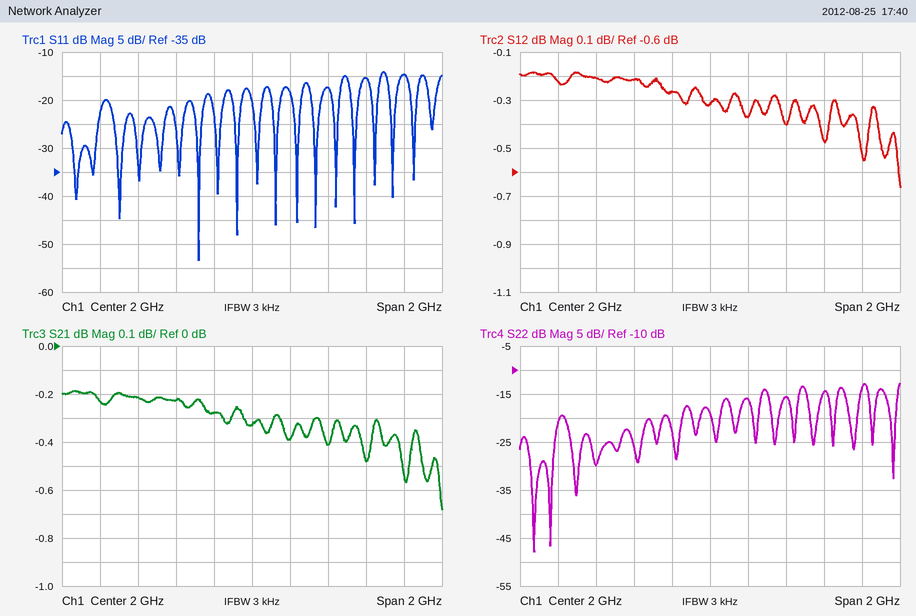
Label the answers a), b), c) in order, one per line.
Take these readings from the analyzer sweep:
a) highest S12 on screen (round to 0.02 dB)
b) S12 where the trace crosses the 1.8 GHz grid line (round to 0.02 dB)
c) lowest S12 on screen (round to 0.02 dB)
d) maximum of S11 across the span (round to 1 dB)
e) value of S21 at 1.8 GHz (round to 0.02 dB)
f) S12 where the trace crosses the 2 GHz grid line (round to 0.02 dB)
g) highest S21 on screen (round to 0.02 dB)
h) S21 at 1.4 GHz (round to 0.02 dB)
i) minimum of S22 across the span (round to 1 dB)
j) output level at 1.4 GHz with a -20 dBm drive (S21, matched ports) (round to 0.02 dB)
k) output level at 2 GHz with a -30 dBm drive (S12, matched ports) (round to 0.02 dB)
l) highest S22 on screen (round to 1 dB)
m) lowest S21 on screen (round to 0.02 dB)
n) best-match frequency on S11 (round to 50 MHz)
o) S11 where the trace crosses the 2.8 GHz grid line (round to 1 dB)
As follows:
a) -0.18 dB
b) -0.26 dB
c) -0.66 dB
d) -14 dB
e) -0.28 dB
f) -0.32 dB
g) -0.18 dB
h) -0.22 dB
i) -48 dB
j) -20.22 dBm
k) -30.32 dBm
l) -13 dB
m) -0.68 dB
n) 1.70 GHz
o) -15 dB
